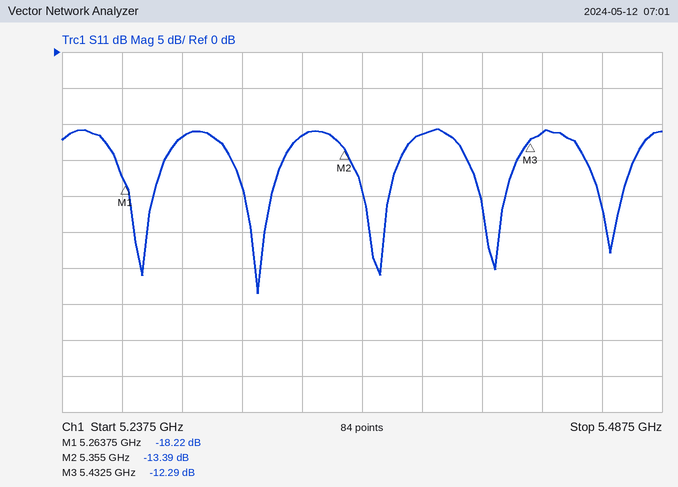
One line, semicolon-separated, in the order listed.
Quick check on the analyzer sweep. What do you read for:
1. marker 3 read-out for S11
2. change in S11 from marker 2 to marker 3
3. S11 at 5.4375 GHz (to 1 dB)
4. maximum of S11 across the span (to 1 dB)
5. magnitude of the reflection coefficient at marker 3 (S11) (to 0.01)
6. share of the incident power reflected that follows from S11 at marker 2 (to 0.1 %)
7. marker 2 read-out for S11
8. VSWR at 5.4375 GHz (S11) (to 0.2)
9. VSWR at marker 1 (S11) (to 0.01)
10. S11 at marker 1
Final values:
-12.29 dB; 1.10 dB; -11 dB; -11 dB; 0.24; 4.6 %; -13.39 dB; 1.8; 1.28; -18.22 dB
